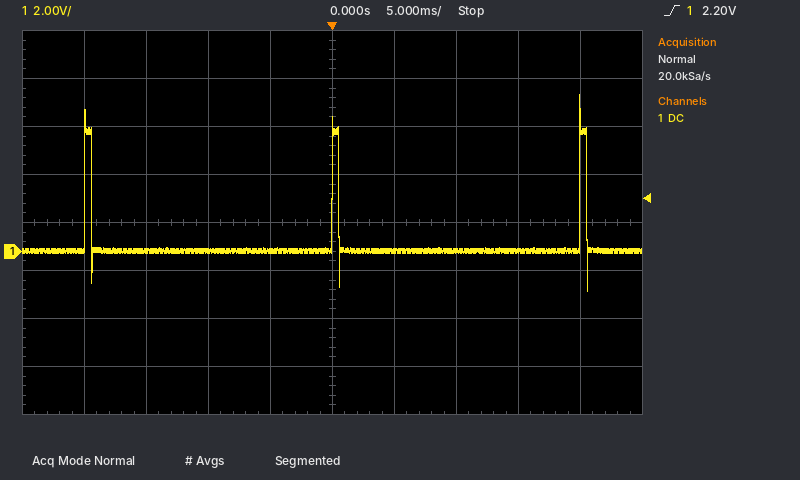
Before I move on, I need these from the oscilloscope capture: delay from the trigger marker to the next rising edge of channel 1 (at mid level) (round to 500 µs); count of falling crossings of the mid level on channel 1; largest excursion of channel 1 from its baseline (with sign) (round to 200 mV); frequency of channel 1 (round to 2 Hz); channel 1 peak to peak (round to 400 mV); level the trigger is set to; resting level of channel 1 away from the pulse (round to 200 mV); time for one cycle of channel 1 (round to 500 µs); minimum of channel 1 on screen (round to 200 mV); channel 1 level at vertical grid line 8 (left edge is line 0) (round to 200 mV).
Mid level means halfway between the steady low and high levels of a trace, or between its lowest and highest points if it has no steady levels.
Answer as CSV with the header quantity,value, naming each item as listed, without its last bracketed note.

quantity,value
delay from the trigger marker to the next rising edge of channel 1 (at mid level),20.0 ms
count of falling crossings of the mid level on channel 1,3
largest excursion of channel 1 from its baseline (with sign),+6.4 V
frequency of channel 1,50 Hz
channel 1 peak to peak,8.0 V
level the trigger is set to,2.20 V
resting level of channel 1 away from the pulse,0.0 V
time for one cycle of channel 1,20.0 ms
minimum of channel 1 on screen,-1.6 V
channel 1 level at vertical grid line 8 (left edge is line 0),0.0 V
